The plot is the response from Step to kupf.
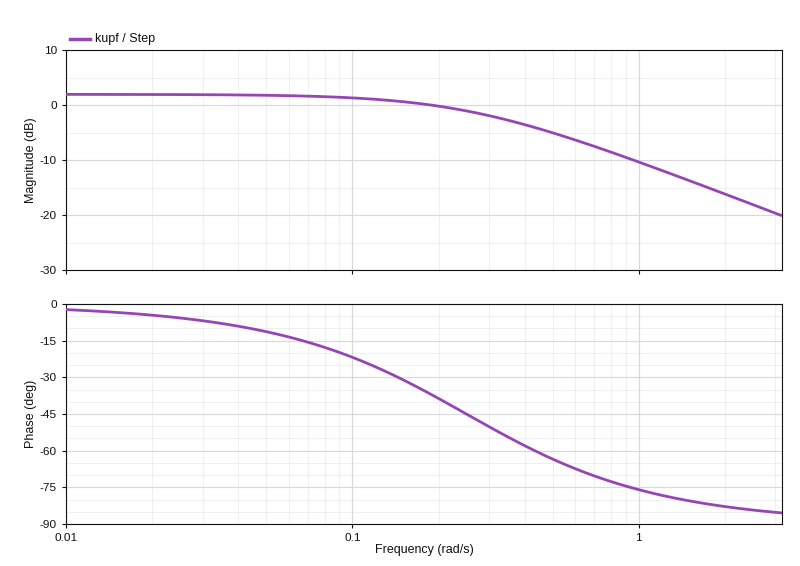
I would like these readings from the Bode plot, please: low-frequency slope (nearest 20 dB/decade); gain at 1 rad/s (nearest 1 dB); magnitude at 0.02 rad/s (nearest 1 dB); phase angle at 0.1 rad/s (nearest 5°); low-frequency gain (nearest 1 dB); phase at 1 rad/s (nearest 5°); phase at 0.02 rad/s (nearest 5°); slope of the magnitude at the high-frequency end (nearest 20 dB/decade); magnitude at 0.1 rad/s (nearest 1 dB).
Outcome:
0 dB/decade
-10 dB
2 dB
-20°
2 dB
-75°
-5°
-20 dB/decade
1 dB
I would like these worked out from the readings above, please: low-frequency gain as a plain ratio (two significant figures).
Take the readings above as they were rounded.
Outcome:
1.3
